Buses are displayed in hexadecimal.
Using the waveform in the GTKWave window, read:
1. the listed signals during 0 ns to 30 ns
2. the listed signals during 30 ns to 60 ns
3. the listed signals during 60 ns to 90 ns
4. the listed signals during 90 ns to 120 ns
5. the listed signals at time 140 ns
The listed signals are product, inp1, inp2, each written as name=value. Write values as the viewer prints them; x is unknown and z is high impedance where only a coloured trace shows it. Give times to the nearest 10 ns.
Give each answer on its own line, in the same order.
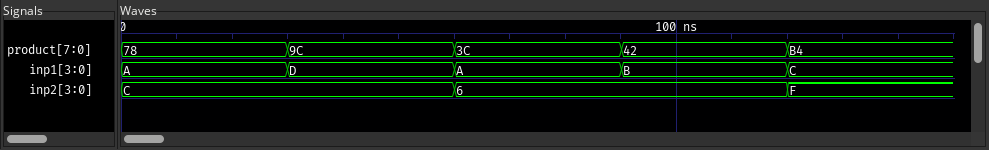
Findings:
product=78, inp1=A, inp2=C
product=9C, inp1=D, inp2=C
product=3C, inp1=A, inp2=6
product=42, inp1=B, inp2=6
product=B4, inp1=C, inp2=F
